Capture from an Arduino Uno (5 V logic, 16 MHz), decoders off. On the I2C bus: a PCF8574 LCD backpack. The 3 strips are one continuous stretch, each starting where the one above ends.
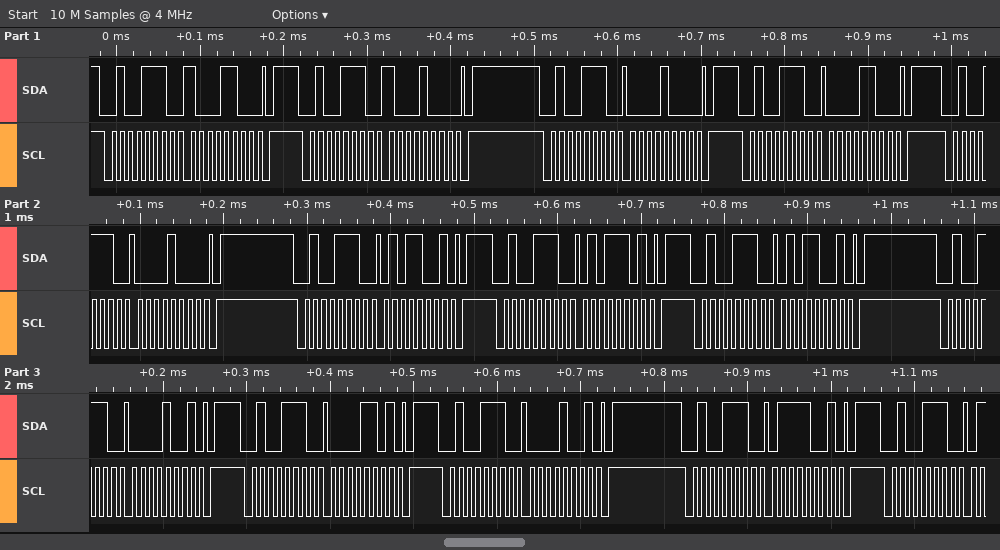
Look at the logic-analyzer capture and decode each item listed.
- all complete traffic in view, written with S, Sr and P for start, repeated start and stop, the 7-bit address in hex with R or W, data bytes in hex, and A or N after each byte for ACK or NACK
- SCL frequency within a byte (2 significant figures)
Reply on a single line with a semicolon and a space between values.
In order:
S 27W A 8C A P S 27W A 88 A P S 27W A 08 A P S 27W A 0C A P S 27W A 08 A P S 27W A 59 A P S 27W A 5D A P S 27W A 59 A P S 27W A 09 A P S 27W A 0D A P S 27W A 09 A P S 27W A 79 A P S 27W A; 100 kHz
